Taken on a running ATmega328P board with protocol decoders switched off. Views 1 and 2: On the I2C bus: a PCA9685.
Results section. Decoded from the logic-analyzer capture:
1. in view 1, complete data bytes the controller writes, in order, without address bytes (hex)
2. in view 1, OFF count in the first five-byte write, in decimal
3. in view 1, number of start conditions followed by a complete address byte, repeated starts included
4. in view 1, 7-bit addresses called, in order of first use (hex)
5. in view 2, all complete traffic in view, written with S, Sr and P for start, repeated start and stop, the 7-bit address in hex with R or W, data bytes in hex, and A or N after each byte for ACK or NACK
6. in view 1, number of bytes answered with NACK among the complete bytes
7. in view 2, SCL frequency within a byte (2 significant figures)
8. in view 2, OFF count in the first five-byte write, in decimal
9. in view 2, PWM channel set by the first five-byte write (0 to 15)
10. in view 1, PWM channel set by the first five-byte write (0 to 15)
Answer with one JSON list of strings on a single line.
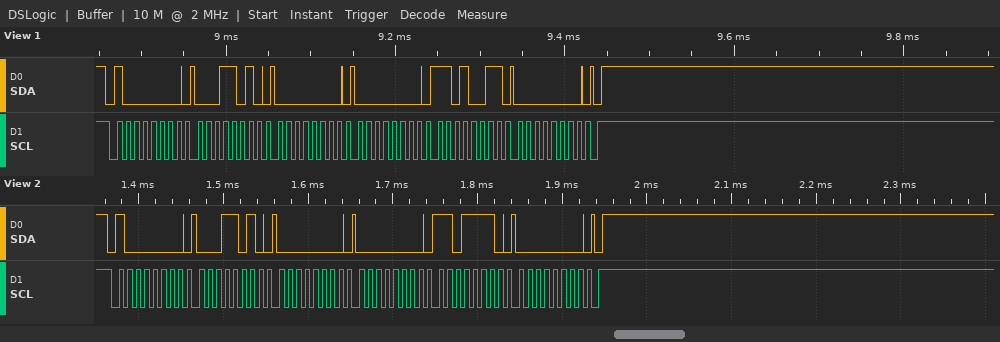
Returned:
["1A 00 00 D3 00", "211", "1", "0x40", "S 40W A 1A A 00 A 00 A DE A 00 A P", "0", "100 kHz", "222", "5", "5"]
